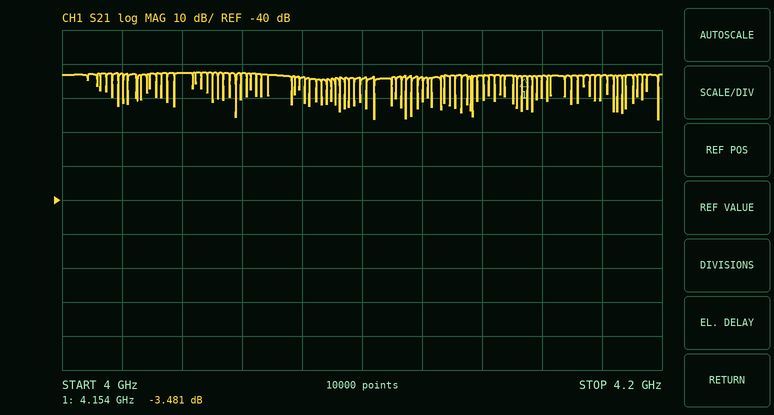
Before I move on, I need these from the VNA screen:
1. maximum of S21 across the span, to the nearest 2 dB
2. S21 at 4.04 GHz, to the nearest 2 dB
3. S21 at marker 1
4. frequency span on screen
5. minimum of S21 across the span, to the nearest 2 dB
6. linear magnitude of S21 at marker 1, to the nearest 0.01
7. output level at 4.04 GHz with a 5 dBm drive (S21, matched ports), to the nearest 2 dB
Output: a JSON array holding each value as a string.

["-2 dB", "-2 dB", "-3.481 dB", "200 MHz", "-16 dB", "0.67", "2 dBm"]
